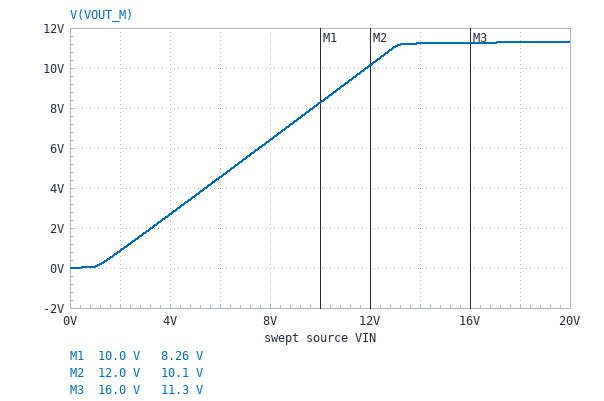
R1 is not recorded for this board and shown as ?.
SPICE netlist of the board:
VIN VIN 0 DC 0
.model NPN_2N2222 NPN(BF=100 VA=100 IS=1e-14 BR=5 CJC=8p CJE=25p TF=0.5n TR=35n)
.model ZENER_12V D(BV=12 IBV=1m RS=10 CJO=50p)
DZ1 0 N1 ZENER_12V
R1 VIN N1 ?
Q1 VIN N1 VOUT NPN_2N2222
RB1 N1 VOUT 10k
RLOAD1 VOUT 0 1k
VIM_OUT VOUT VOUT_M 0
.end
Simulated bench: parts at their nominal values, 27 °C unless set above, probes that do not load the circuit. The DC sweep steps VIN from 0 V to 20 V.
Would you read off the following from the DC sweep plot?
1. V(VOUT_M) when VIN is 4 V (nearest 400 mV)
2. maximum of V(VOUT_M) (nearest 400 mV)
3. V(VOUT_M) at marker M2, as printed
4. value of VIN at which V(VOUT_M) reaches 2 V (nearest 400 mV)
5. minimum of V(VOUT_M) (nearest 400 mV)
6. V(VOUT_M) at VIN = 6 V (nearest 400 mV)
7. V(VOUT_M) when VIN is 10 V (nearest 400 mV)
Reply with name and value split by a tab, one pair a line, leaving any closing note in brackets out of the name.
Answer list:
V(VOUT_M) when VIN is 4 V	2.8 V
maximum of V(VOUT_M)	11.2 V
V(VOUT_M) at marker M2, as printed	10.1 V
value of VIN at which V(VOUT_M) reaches 2 V	3.2 V
minimum of V(VOUT_M)	0 V
V(VOUT_M) at VIN = 6 V	4.4 V
V(VOUT_M) when VIN is 10 V	8.4 V
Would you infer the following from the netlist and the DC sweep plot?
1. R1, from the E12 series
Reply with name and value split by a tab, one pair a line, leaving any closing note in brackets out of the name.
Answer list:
R1, from the E12 series	6.8 kΩ
